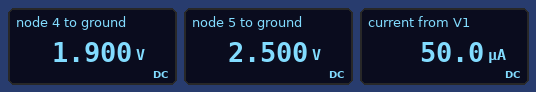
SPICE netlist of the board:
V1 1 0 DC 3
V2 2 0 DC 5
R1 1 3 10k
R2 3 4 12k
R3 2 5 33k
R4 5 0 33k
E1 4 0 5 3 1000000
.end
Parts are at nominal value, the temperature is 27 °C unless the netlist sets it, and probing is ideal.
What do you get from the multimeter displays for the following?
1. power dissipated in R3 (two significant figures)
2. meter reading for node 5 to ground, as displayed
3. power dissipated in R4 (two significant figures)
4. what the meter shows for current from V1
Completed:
190 µW
2.500 V
190 µW
50.0 µA
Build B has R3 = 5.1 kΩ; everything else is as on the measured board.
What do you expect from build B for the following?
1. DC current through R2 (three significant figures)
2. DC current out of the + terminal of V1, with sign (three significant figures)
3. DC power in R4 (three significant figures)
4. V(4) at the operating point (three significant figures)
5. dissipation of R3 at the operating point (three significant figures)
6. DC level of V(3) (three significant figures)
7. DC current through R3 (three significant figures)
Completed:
133 µA
-133 µA
568 µW
5.93 V
87.8 µW
4.33 V
131 µA
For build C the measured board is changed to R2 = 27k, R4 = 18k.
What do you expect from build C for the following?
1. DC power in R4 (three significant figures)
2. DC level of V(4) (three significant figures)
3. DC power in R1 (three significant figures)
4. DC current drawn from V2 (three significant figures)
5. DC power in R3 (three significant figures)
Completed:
173 µW
-1.57 V
153 µW
98.0 µA
317 µW
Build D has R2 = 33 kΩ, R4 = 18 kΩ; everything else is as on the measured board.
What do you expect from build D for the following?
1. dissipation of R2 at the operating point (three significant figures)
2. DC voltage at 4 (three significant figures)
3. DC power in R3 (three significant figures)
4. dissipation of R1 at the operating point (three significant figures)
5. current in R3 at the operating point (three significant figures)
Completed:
504 µW
-2.31 V
317 µW
153 µW
98.0 µA
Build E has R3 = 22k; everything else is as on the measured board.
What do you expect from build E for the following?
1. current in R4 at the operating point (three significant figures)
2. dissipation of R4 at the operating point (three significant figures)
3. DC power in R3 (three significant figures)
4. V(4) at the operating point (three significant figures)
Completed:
90.9 µA
273 µW
182 µW
3.00 V
